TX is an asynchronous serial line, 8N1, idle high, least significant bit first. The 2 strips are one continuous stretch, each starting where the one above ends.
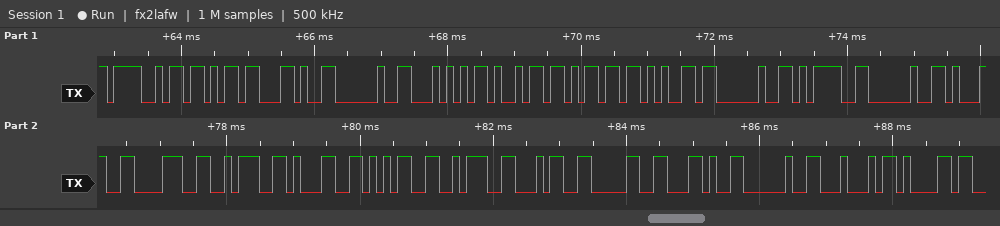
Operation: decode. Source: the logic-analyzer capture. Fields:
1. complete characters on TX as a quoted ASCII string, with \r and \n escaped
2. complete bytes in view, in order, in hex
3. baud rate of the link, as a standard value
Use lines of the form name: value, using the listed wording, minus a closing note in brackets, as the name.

complete characters on TX as a quoted ASCII string, with \r and \n escaped: "Ok, Time = 18:15:40, Da"
complete bytes in view, in order, in hex: 4F 6B 2C 20 54 69 6D 65 20 3D 20 31 38 3A 31 35 3A 34 30 2C 20 44 61
baud rate of the link, as a standard value: 9600 baud
